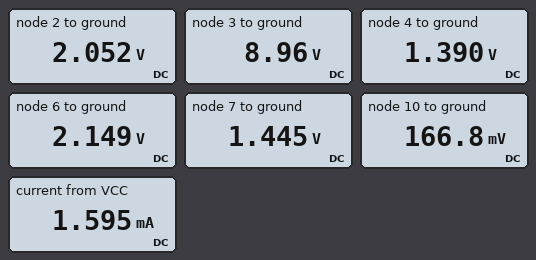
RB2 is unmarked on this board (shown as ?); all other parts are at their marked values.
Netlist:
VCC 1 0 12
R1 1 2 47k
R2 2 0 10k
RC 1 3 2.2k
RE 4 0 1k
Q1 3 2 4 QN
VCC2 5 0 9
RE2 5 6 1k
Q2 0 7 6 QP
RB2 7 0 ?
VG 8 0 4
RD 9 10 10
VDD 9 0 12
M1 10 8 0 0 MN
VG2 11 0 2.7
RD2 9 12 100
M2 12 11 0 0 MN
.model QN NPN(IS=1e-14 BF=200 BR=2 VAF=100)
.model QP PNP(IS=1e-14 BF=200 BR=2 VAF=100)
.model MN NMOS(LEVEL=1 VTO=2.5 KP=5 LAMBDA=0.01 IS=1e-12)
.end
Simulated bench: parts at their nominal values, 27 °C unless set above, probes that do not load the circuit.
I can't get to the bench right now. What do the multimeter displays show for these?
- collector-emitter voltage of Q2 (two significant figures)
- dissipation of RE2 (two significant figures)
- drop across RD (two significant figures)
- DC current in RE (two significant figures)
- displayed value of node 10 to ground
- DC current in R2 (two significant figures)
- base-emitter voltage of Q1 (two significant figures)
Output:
-2.1 V
47 mW
12 V
1.4 mA
166.8 mV
210 µA
660 mV
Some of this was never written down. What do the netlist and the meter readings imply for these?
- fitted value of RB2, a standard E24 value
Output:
43 kΩ
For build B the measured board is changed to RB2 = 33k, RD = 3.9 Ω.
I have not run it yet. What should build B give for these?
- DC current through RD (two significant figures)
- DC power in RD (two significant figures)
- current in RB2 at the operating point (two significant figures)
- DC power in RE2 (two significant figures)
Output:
3.0 A
34 W
35 µA
51 mW
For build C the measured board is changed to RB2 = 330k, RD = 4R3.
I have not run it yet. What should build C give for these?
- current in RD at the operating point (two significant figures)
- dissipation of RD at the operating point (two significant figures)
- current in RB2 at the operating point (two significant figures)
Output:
2.7 A
31 W
15 µA
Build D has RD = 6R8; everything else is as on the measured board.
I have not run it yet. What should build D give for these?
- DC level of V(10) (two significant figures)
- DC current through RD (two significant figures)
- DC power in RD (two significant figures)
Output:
250 mV
1.7 A
20 W
